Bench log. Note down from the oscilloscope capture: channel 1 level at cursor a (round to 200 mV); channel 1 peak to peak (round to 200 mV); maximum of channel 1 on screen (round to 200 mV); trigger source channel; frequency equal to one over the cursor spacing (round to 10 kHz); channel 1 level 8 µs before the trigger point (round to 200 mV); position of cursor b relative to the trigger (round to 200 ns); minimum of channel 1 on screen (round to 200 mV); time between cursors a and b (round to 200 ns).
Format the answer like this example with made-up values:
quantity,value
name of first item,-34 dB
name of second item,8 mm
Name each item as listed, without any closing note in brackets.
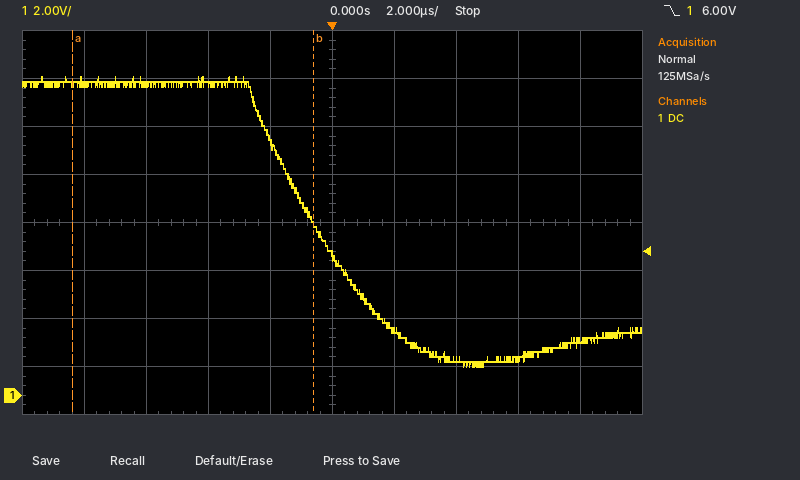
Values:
quantity,value
channel 1 level at cursor a,13.0 V
channel 1 peak to peak,12.0 V
maximum of channel 1 on screen,13.2 V
trigger source channel,channel 1
frequency equal to one over the cursor spacing,130 kHz
channel 1 level 8 µs before the trigger point,13.0 V
position of cursor b relative to the trigger,-600 ns
minimum of channel 1 on screen,1.2 V
time between cursors a and b,7.8 µs
